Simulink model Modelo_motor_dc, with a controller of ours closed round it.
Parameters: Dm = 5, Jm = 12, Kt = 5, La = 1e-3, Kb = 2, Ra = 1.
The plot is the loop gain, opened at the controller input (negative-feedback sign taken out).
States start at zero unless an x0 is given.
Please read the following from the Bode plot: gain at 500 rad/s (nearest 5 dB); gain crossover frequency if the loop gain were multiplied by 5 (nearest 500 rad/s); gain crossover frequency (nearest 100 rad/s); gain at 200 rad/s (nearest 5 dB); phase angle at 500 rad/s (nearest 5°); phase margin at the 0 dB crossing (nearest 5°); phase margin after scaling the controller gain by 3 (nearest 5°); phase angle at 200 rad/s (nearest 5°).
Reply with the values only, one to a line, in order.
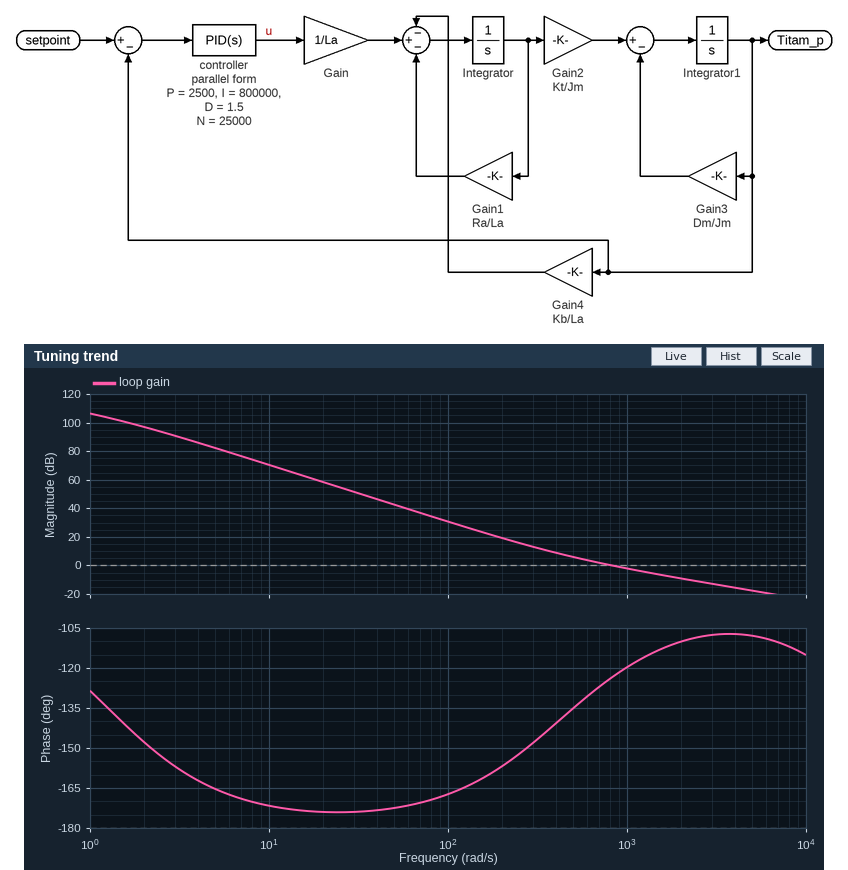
5 dB
3500 rad/s
800 rad/s
20 dB
-135°
55°
70°
-155°
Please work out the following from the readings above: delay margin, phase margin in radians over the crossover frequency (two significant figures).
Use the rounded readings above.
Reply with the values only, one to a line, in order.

0.0012 s
